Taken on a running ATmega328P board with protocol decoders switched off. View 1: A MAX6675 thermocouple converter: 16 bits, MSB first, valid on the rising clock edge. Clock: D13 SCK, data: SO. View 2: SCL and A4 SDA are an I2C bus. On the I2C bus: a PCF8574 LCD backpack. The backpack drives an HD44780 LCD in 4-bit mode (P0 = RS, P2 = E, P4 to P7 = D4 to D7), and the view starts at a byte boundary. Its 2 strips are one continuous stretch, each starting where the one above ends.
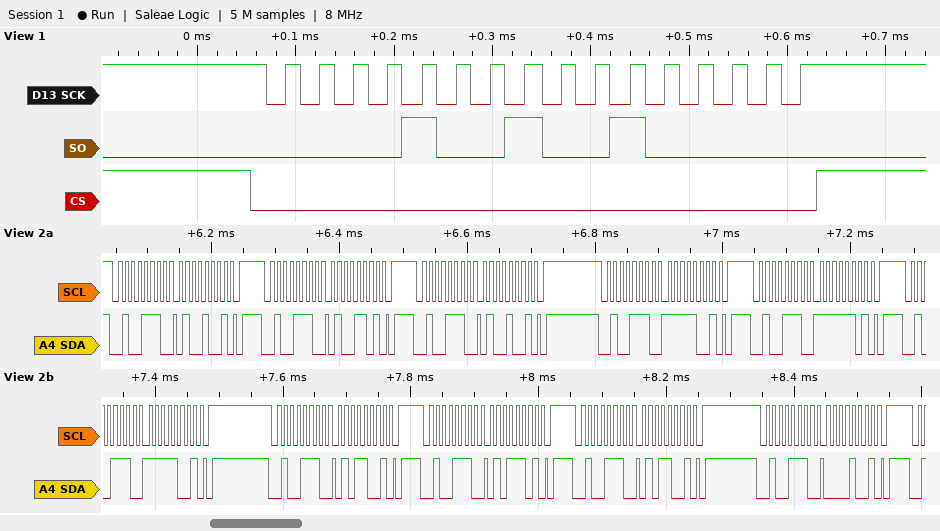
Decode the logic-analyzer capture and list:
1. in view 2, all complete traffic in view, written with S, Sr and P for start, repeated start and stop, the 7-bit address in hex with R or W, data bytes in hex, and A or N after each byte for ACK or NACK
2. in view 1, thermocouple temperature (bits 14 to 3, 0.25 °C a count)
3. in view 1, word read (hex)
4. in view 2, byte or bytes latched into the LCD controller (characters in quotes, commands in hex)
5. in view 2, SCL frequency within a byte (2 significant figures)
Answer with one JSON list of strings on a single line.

["S 27W A 49 A P S 27W A 4D A P S 27W A 49 A P S 27W A F9 A P S 27W A FD A P S 27W A F9 A P S 27W A 59 A P S 27W A 5D A P S 27W A 59 A P S 27W A 09 A P", "73.00 °C", "0x0920", "'O'", "100 kHz"]
